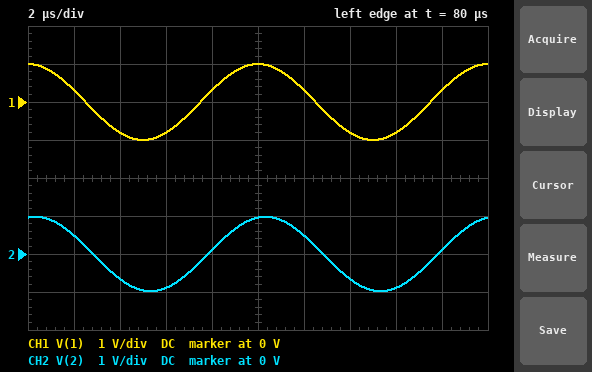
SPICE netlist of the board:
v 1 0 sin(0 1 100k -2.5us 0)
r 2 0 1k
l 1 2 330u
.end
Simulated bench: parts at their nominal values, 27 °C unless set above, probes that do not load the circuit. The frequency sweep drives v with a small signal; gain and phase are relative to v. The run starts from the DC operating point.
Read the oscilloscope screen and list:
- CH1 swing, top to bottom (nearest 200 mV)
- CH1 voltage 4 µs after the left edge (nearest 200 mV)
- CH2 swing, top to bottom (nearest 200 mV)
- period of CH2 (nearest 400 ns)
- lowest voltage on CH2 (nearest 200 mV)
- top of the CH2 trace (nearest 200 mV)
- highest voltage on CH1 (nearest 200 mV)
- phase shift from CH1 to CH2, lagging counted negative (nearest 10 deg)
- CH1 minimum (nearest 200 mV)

2.0 V
-800 mV
2.0 V
10.0 µs
-1.0 V
1.0 V
1.0 V
-10 deg
-1.0 V
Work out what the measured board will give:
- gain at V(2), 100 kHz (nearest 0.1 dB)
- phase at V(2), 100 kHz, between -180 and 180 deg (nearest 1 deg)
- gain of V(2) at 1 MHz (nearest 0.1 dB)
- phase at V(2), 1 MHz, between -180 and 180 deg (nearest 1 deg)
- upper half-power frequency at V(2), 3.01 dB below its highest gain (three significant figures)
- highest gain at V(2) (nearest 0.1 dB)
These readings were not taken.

-0.2 dB
-12 deg
-7.2 dB
-64 deg
482 kHz
0 dB
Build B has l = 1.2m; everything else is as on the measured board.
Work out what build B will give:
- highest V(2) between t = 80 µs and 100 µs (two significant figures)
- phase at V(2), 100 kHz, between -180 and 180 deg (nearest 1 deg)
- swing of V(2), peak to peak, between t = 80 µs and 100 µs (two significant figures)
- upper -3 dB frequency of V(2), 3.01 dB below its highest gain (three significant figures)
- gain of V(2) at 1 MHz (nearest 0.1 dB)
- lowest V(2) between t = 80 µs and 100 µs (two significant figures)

800 mV
-37 deg
1.6 V
133 kHz
-17.6 dB
-800 mV
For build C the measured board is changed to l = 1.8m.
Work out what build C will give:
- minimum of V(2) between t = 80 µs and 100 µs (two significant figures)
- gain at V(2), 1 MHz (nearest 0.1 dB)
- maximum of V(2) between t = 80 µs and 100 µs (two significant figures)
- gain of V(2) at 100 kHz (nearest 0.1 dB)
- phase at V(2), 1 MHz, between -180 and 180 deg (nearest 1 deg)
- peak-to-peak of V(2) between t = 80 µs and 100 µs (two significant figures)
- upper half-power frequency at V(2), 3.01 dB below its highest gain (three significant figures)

-660 mV
-21.1 dB
660 mV
-3.6 dB
-85 deg
1.3 V
88.4 kHz
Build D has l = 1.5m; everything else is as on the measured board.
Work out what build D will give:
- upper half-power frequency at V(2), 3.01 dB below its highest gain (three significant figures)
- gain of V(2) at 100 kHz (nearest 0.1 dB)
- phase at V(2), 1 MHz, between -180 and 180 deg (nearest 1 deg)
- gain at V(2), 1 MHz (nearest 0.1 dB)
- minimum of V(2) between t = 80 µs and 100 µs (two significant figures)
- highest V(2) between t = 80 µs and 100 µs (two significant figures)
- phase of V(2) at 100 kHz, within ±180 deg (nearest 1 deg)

106 kHz
-2.8 dB
-84 deg
-19.5 dB
-730 mV
730 mV
-43 deg
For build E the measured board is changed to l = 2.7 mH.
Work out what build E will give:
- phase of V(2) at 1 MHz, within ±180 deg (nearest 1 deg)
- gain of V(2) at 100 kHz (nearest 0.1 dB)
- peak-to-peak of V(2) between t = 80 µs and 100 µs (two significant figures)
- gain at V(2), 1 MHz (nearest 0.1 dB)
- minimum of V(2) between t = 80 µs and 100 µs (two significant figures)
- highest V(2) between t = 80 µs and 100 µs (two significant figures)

-87 deg
-5.9 dB
1.0 V
-24.6 dB
-510 mV
510 mV
